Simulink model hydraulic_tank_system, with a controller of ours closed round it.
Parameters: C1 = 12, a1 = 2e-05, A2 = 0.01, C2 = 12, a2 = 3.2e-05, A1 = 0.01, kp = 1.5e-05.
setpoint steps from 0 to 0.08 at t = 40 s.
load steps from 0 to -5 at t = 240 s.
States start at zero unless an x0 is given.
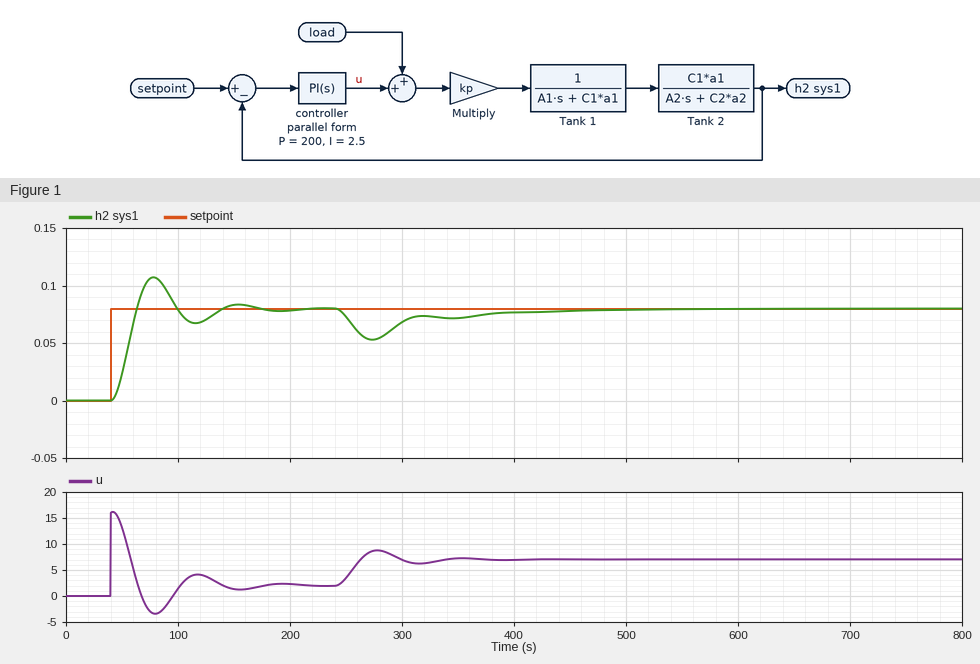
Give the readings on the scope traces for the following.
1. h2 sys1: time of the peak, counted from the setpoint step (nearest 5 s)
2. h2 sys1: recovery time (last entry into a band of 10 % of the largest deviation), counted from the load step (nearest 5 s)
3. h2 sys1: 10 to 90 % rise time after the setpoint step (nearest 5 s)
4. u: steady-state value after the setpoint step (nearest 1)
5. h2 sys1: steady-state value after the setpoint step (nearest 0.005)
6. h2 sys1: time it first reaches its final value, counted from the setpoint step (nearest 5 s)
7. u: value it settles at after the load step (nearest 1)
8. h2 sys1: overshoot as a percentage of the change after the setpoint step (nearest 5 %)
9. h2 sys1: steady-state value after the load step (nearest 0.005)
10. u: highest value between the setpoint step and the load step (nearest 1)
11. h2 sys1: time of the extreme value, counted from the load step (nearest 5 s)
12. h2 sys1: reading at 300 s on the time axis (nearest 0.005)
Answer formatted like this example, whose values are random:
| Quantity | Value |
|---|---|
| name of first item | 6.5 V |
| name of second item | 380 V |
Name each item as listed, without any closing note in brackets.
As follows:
| Quantity | Value |
|---|---|
| h2 sys1: time of the peak, counted from the setpoint step | 40 s |
| h2 sys1: recovery time (last entry into a band of 10 % of the largest deviation), counted from the load step | 195 s |
| h2 sys1: 10 to 90 % rise time after the setpoint step | 15 s |
| u: steady-state value after the setpoint step | 2 |
| h2 sys1: steady-state value after the setpoint step | 0.080 |
| h2 sys1: time it first reaches its final value, counted from the setpoint step | 25 s |
| u: value it settles at after the load step | 7 |
| h2 sys1: overshoot as a percentage of the change after the setpoint step | 35 % |
| h2 sys1: steady-state value after the load step | 0.080 |
| u: highest value between the setpoint step and the load step | 16 |
| h2 sys1: time of the extreme value, counted from the load step | 35 s |
| h2 sys1: reading at 300 s on the time axis | 0.070 |
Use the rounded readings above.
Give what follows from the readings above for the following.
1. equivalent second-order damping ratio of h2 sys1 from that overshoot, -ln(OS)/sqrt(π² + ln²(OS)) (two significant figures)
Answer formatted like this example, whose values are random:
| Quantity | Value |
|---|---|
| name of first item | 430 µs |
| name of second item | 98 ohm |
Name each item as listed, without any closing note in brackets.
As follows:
| Quantity | Value |
|---|---|
| equivalent second-order damping ratio of h2 sys1 from that overshoot, -ln(OS)/sqrt(π² + ln²(OS)) | 0.32 |
